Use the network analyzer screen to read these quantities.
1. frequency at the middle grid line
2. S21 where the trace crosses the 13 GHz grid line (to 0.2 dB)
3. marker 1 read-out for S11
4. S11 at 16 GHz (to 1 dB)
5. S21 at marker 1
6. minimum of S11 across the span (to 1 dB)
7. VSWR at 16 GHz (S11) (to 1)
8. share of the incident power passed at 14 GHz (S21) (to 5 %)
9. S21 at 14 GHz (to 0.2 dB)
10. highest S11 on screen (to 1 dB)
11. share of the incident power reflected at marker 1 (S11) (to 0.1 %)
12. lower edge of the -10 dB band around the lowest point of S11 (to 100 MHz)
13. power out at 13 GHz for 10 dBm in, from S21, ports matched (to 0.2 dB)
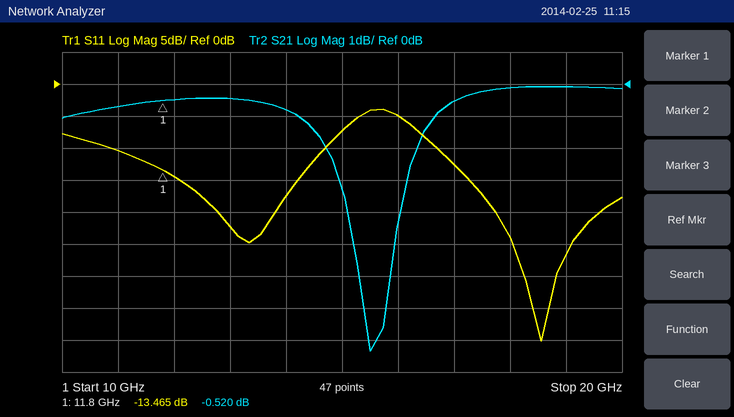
15 GHz
-0.4 dB
-13.465 dB
-5 dB
-0.520 dB
-40 dB
4
85 %
-0.8 dB
-4 dB
4.5 %
16.7 GHz
9.6 dBm
